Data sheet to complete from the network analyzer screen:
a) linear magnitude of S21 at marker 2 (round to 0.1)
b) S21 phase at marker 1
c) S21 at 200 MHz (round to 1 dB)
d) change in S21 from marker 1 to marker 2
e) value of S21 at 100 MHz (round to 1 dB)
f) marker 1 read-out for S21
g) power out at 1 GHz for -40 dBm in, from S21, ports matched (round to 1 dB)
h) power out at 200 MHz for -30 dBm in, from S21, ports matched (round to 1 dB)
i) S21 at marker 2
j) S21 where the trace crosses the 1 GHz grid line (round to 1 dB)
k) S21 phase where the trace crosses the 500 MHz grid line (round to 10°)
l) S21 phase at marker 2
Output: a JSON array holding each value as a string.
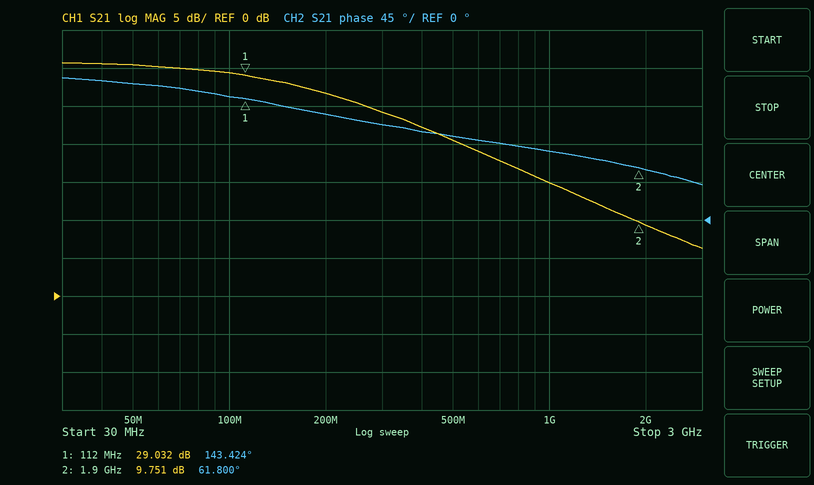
["3.1", "143.424°", "27 dB", "-19.281 dB", "29 dB", "29.032 dB", "-25 dBm", "-3 dBm", "9.751 dB", "15 dB", "100°", "61.800°"]
